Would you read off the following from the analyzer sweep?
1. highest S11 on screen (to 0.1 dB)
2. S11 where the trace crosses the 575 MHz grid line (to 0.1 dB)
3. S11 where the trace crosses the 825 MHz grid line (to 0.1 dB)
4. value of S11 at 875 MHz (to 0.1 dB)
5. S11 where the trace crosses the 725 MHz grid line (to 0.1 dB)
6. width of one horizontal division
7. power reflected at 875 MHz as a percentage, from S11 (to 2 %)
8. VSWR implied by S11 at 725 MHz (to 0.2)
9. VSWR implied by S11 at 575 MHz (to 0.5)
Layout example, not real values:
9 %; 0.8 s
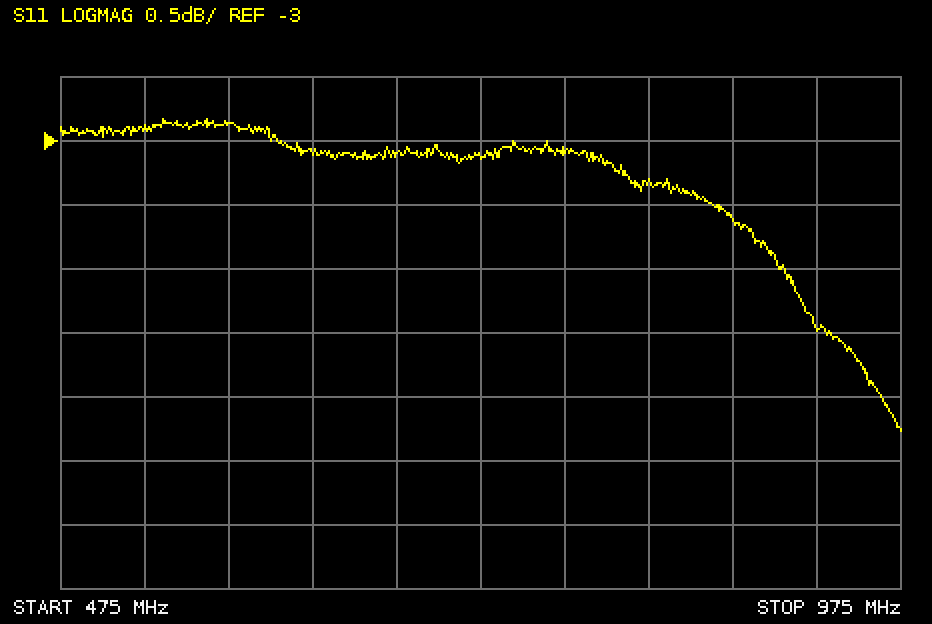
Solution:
-2.8 dB; -2.9 dB; -3.3 dB; -3.6 dB; -3.1 dB; 50 MHz; 44 %; 5.6; 6.0
